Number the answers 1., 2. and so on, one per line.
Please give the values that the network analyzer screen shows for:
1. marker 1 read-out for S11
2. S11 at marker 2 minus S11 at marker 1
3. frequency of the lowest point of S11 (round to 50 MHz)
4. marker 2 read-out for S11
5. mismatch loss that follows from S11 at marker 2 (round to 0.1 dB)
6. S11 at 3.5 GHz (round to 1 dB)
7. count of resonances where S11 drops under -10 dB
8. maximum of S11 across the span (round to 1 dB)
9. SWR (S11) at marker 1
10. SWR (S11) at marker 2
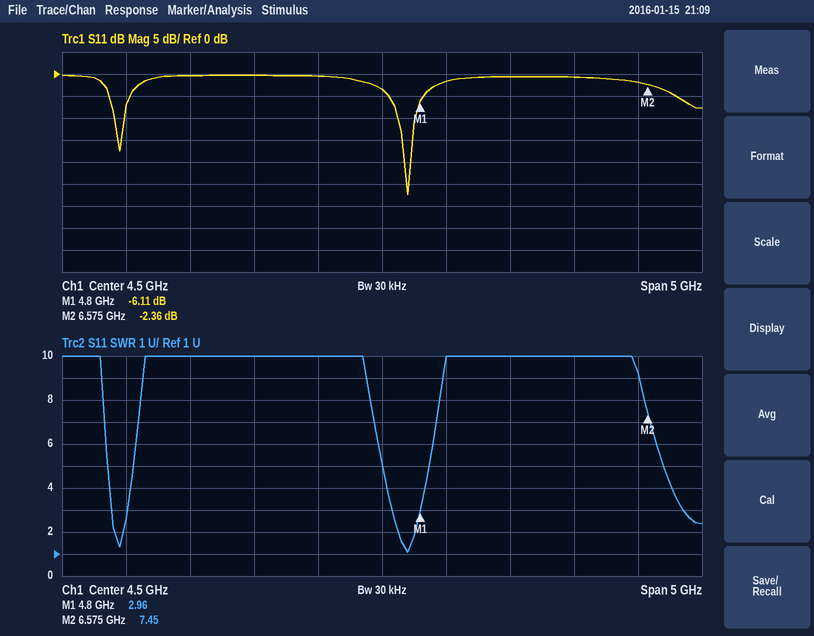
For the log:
1. -6.11 dB
2. 3.75 dB
3. 4.70 GHz
4. -2.36 dB
5. 3.8 dB
6. 0 dB
7. 2
8. 0 dB
9. 2.96
10. 7.45
